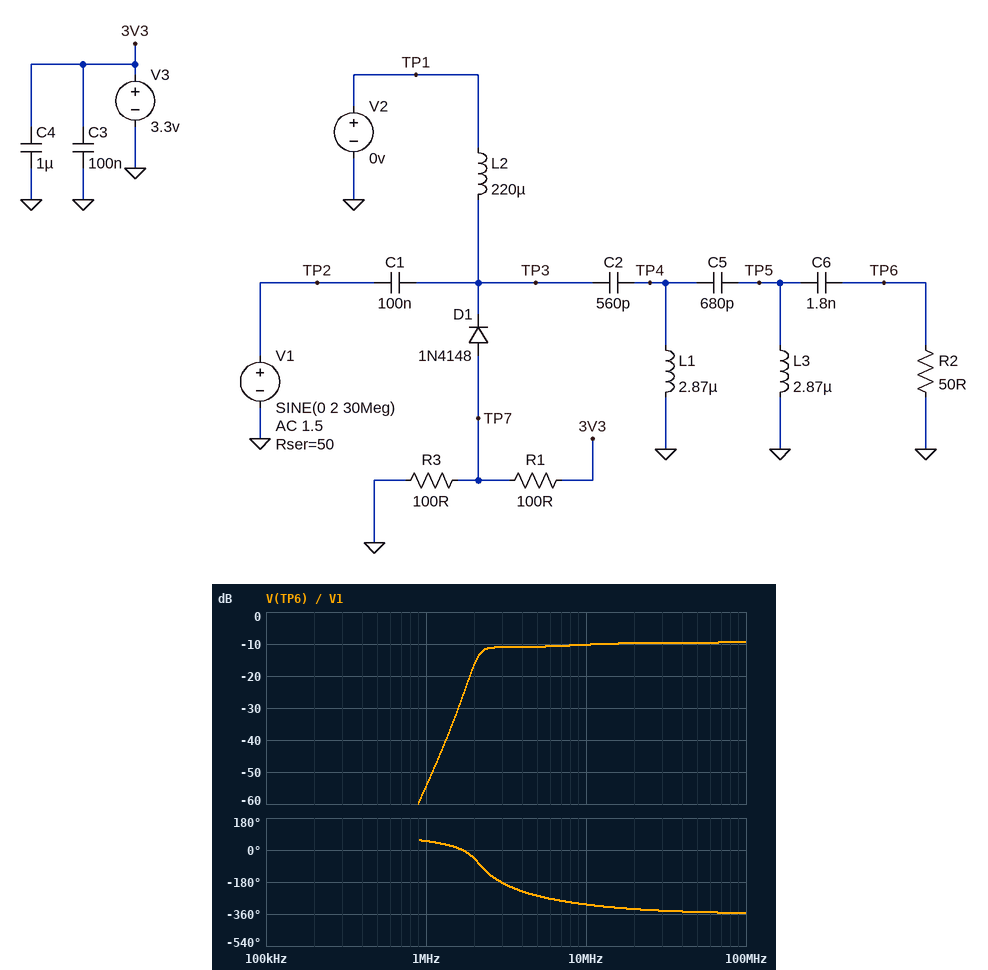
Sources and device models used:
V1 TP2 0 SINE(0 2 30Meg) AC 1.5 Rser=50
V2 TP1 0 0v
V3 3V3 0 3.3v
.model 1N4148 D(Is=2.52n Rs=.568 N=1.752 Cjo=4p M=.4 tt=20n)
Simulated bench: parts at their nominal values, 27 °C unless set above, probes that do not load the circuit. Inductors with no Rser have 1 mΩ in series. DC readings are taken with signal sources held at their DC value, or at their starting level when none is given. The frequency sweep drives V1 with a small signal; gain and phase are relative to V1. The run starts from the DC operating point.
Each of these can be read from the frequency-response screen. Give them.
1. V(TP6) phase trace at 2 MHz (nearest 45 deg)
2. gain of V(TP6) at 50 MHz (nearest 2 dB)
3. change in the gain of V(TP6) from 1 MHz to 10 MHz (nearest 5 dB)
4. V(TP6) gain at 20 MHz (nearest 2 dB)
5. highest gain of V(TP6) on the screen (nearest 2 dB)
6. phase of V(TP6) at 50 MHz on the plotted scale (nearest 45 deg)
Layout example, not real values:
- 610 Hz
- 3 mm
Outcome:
- -45 deg
- -10 dB
- 45 dB
- -10 dB
- -10 dB
- -360 deg
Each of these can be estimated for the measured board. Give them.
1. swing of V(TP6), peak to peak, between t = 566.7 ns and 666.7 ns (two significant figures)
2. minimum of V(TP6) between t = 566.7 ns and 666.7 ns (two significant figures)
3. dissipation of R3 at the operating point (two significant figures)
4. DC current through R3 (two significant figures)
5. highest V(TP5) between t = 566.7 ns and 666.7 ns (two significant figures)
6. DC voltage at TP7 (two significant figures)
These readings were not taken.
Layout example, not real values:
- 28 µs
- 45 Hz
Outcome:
- 1.3 V
- -660 mV
- 5.3 mW
- 7.3 mA
- 670 mV
- 730 mV
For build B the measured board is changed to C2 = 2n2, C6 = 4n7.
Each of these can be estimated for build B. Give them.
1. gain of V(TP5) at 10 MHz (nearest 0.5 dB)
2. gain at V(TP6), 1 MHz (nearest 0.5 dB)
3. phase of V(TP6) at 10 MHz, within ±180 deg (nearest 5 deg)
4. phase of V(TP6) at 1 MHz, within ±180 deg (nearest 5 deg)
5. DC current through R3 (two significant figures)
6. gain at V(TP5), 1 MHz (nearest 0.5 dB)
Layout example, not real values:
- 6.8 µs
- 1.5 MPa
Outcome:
- -9.5 dB
- -37.0 dB
- 35 deg
- -10 deg
- 7.3 mA
- -35.5 dB
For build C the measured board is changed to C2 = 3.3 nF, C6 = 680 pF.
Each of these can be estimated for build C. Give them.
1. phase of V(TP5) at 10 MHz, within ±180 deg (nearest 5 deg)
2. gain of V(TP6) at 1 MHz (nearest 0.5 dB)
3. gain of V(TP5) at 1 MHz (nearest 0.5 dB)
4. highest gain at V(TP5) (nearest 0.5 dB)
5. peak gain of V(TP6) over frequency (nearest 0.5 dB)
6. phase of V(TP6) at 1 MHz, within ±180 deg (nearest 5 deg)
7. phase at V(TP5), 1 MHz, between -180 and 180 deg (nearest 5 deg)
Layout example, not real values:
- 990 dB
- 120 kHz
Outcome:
- 20 deg
- -46.0 dB
- -32.5 dB
- -3.0 dB
- -9.0 dB
- 35 deg
- -40 deg
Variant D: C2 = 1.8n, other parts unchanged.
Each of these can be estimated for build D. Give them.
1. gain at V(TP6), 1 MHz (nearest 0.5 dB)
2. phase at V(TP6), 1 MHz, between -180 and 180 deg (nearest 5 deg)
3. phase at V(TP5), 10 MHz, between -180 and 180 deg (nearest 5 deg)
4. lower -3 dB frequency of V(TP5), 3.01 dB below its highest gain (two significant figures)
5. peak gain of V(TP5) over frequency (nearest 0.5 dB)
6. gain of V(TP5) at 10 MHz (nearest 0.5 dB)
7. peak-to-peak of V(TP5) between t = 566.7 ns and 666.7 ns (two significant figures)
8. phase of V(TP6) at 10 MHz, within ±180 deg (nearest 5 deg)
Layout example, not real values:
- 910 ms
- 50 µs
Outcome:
- -43.5 dB
- 35 deg
- 30 deg
- 1.7 MHz
- -7.5 dB
- -9.5 dB
- 1.3 V
- 40 deg
